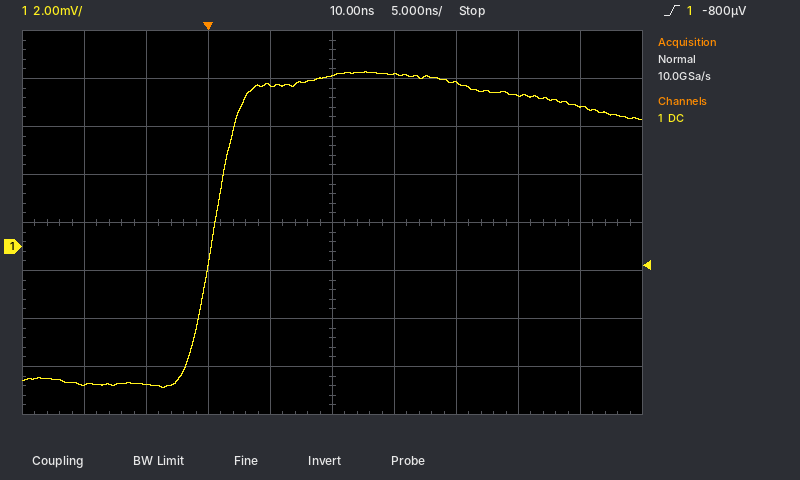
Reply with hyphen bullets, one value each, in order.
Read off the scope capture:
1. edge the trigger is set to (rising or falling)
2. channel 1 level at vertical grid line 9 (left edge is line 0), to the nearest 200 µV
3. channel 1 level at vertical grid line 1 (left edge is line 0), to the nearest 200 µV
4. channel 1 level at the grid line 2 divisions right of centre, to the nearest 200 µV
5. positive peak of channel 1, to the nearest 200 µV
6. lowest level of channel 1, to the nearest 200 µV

- rising
- 5.8 mV
- -5.8 mV
- 6.8 mV
- 7.2 mV
- -5.8 mV
